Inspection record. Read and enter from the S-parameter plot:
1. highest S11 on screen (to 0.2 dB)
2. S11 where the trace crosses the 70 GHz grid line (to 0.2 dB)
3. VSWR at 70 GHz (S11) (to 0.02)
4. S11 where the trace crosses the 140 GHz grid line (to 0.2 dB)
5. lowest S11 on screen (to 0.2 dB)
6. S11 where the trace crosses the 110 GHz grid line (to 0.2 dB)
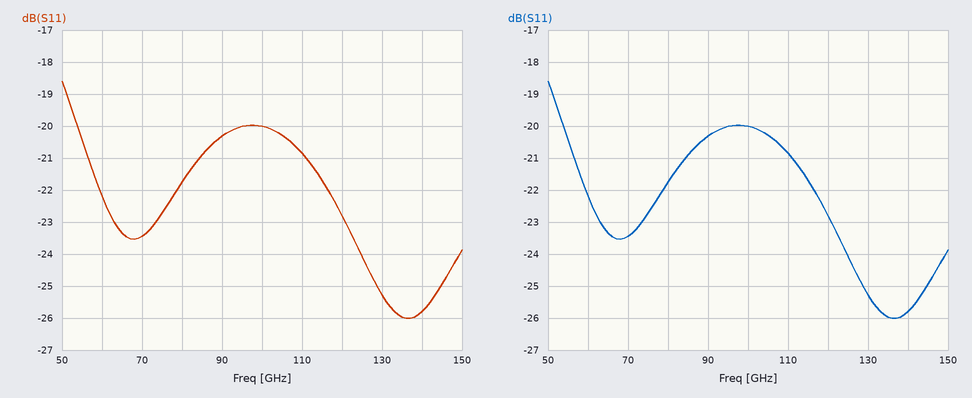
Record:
-18.6 dB
-23.4 dB
1.14
-25.8 dB
-26.0 dB
-20.8 dB
